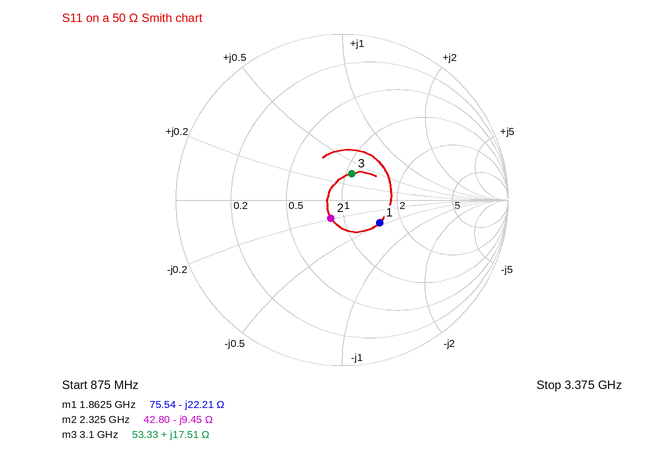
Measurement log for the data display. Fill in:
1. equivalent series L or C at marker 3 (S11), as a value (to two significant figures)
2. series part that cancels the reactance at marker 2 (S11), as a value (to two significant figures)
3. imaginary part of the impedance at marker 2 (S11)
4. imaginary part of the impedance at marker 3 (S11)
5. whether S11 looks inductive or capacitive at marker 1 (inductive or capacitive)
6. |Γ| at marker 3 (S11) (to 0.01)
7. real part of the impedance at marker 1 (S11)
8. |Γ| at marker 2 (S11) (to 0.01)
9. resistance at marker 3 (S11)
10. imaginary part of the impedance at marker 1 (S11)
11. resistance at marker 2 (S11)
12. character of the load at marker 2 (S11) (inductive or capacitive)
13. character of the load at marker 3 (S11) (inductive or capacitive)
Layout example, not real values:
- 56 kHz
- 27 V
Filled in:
- 900 pH
- 650 pH
- -9.45 Ω
- +17.51 Ω
- capacitive
- 0.17
- 75.54 Ω
- 0.13
- 53.33 Ω
- -22.21 Ω
- 42.80 Ω
- capacitive
- inductive
